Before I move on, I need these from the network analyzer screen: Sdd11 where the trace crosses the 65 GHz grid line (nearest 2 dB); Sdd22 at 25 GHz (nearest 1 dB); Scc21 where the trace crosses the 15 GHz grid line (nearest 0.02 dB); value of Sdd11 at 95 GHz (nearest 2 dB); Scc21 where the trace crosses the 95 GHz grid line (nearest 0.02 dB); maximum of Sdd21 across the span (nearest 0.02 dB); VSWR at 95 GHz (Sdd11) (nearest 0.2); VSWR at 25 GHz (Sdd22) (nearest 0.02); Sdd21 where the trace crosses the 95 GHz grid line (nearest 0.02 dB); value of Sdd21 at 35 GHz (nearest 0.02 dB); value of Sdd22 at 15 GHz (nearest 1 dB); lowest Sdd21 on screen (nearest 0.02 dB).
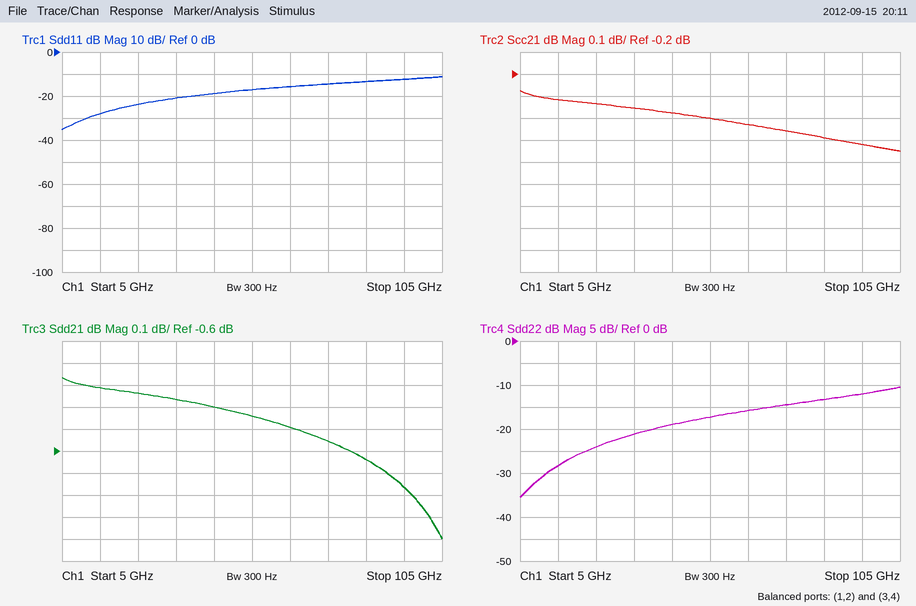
-16 dB
-24 dB
-0.32 dB
-12 dB
-0.52 dB
-0.26 dB
1.6
1.14
-0.76 dB
-0.36 dB
-28 dB
-1.00 dB
